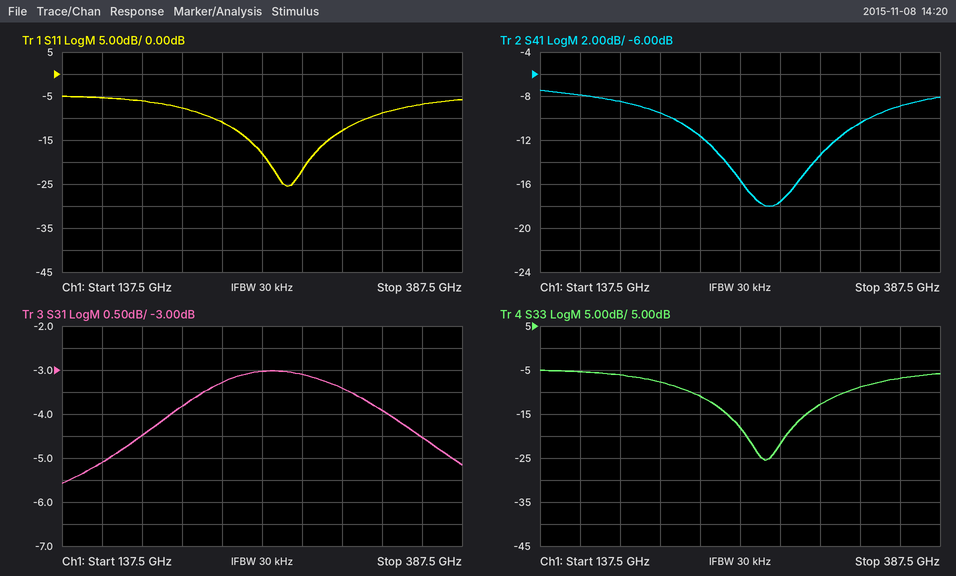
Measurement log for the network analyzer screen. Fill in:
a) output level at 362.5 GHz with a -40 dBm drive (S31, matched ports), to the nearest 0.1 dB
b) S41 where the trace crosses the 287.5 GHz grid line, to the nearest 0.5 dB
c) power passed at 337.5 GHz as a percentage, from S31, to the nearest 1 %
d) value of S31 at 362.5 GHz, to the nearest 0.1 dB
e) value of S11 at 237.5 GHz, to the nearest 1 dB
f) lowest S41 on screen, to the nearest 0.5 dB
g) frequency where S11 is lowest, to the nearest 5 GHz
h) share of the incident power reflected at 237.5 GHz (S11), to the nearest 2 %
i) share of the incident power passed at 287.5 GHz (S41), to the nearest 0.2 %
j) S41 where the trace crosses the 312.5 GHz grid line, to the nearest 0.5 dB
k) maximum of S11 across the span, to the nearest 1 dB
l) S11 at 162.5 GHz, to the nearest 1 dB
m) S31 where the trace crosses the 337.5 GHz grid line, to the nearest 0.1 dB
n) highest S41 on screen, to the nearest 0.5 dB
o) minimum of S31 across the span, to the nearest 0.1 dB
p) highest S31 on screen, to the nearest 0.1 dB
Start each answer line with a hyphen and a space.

- -44.5 dBm
- -17.5 dB
- 41 %
- -4.5 dB
- -11 dB
- -18.0 dB
- 280 GHz
- 8 %
- 1.8 %
- -13.5 dB
- -5 dB
- -5 dB
- -3.9 dB
- -7.5 dB
- -5.6 dB
- -3.0 dB
